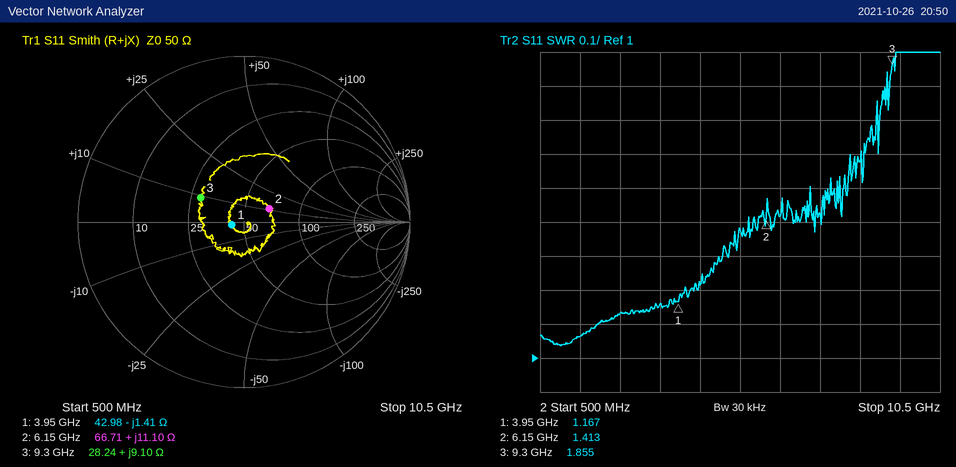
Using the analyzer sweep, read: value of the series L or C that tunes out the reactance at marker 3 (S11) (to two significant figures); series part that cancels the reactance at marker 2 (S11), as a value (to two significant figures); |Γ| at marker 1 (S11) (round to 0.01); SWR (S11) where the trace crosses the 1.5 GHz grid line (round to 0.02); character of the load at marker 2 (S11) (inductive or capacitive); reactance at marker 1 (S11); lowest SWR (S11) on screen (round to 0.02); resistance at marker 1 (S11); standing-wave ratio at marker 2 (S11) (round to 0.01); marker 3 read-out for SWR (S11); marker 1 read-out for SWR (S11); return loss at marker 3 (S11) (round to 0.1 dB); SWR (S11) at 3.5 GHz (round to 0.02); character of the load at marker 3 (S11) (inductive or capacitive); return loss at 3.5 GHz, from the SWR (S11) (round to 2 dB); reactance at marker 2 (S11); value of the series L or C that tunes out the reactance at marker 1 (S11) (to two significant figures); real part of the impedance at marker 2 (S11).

1.9 pF
2.3 pF
0.08
1.06
inductive
-1.41 Ω
1.04
42.98 Ω
1.41
1.855
1.167
10.5 dB
1.16
inductive
22 dB
+11.10 Ω
57 pH
66.71 Ω
